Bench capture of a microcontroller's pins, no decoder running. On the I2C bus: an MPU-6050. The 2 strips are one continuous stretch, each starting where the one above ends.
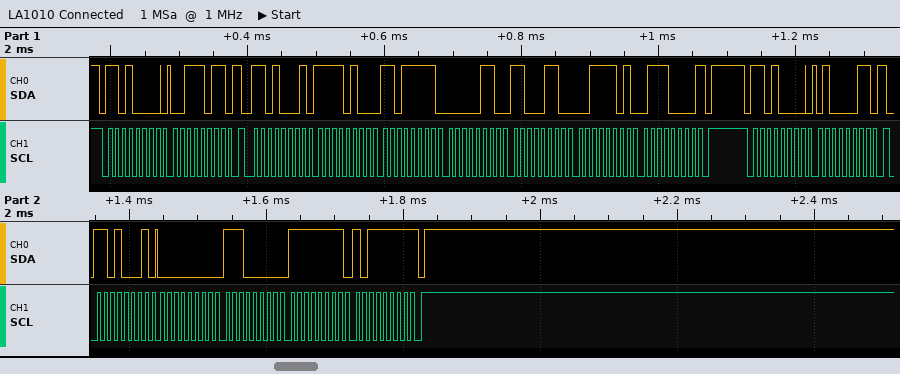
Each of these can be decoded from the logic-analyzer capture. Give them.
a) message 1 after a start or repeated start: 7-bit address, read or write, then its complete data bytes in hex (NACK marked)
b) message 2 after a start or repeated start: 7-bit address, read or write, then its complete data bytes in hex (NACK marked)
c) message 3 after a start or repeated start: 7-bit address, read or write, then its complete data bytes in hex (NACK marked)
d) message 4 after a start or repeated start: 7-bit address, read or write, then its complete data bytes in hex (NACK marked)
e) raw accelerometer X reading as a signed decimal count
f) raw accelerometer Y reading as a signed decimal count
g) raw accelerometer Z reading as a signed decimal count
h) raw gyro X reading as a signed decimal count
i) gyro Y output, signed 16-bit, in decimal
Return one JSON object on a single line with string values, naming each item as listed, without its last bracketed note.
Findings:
{"message 1 after a start or repeated start: 7-bit address, read or write, then its complete data bytes in hex": "0x68 write: 3B", "message 2 after a start or repeated start: 7-bit address, read or write, then its complete data bytes in hex": "0x68 read: F4 DF 06 C6 3D 70 NACK", "message 3 after a start or repeated start: 7-bit address, read or write, then its complete data bytes in hex": "0x68 write: 43", "message 4 after a start or repeated start: 7-bit address, read or write, then its complete data bytes in hex": "0x68 read: 00 E0 FF BF NACK", "raw accelerometer X reading as a signed decimal count": "-2849", "raw accelerometer Y reading as a signed decimal count": "1734", "raw accelerometer Z reading as a signed decimal count": "15728", "raw gyro X reading as a signed decimal count": "224", "gyro Y output, signed 16-bit, in decimal": "-65"}
